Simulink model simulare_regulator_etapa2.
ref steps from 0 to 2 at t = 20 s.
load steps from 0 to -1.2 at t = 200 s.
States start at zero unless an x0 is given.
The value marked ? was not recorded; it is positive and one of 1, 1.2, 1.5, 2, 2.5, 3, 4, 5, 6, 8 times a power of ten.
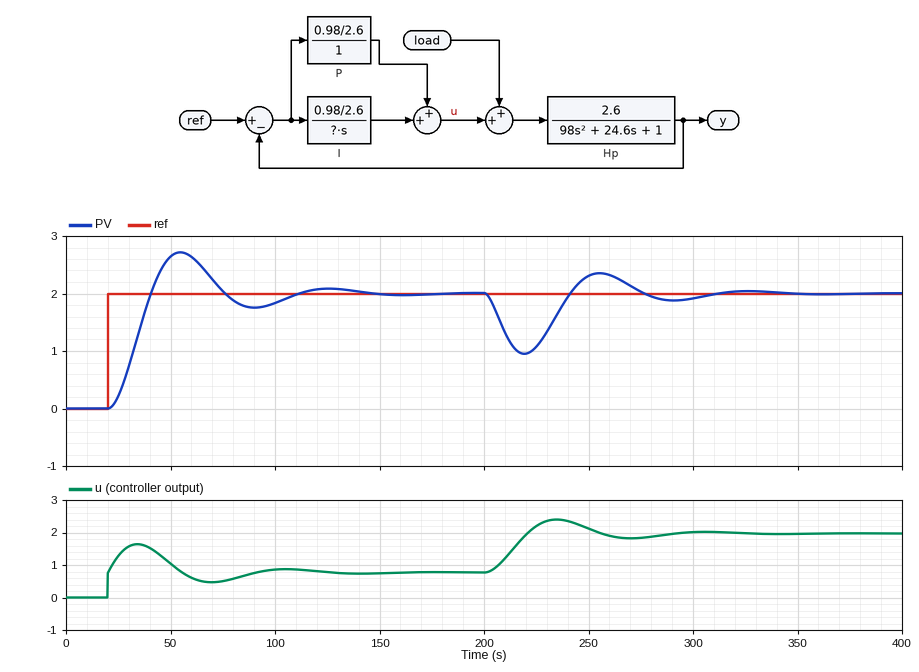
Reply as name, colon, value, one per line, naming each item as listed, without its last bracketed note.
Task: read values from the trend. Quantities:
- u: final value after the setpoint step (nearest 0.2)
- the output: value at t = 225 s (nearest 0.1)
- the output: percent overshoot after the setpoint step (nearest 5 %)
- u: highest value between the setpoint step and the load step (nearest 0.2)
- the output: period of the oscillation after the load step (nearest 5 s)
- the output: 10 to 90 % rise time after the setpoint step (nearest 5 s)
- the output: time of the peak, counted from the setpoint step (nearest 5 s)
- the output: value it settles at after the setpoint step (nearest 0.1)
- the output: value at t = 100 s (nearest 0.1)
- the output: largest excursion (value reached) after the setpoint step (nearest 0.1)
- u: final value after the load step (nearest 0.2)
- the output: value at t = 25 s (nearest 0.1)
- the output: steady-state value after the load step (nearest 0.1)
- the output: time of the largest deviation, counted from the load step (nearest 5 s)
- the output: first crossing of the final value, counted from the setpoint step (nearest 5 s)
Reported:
u: final value after the setpoint step: 0.8
the output: value at t = 225 s: 1.1
the output: percent overshoot after the setpoint step: 35 %
u: highest value between the setpoint step and the load step: 1.6
the output: period of the oscillation after the load step: 70 s
the output: 10 to 90 % rise time after the setpoint step: 15 s
the output: time of the peak, counted from the setpoint step: 35 s
the output: value it settles at after the setpoint step: 2.0
the output: value at t = 100 s: 1.8
the output: largest excursion (value reached) after the setpoint step: 2.7
u: final value after the load step: 2.0
the output: value at t = 25 s: 0.2
the output: steady-state value after the load step: 2.0
the output: time of the largest deviation, counted from the load step: 20 s
the output: first crossing of the final value, counted from the setpoint step: 20 s
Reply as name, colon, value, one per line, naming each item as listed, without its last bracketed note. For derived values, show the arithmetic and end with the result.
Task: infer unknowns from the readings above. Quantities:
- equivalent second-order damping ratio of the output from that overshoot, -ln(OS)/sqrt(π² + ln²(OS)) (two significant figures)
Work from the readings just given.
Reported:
equivalent second-order damping ratio of the output from that overshoot, -ln(OS)/sqrt(π² + ln²(OS)): ln(0.35) = -1.050; 1.050 / sqrt(9.870 + 1.102) = 0.32
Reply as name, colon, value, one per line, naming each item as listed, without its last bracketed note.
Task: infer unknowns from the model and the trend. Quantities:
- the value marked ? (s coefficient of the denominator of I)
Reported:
the value marked ?: 6
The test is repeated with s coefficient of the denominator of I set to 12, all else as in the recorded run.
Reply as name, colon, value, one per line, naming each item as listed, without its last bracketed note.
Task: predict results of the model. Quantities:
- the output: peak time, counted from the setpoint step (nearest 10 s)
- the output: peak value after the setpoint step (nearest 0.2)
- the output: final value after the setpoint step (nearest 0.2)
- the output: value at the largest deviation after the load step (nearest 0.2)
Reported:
the output: peak time, counted from the setpoint step: 50 s
the output: peak value after the setpoint step: 2.2
the output: final value after the setpoint step: 2.0
the output: value at the largest deviation after the load step: 0.8
